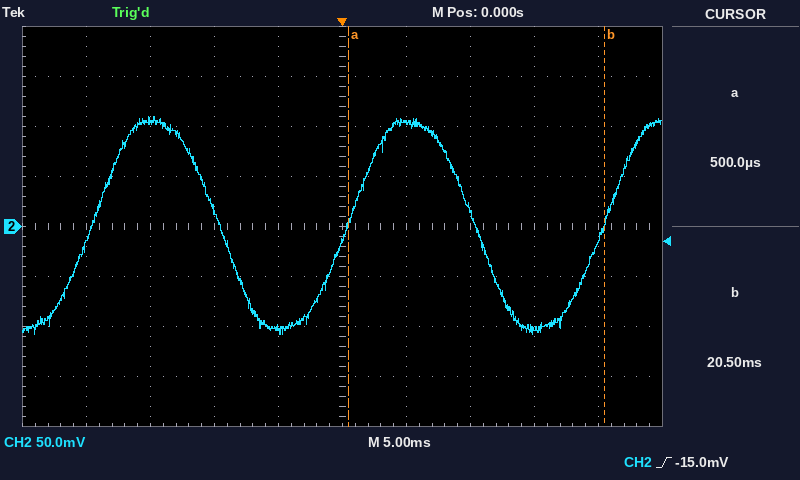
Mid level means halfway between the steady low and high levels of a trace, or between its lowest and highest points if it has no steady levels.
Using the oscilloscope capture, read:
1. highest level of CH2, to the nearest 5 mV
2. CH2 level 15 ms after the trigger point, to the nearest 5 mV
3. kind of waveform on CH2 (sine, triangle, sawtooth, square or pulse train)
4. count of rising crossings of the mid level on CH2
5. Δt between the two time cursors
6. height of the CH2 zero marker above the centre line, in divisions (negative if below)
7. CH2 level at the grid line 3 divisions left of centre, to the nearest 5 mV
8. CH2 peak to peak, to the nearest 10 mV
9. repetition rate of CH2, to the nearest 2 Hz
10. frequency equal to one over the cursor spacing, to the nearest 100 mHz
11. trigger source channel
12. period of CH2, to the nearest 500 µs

110 mV
-105 mV
sine
3
20.0 ms
0.0 div
105 mV
220 mV
50 Hz
50.0 Hz
CH2
20.0 ms
